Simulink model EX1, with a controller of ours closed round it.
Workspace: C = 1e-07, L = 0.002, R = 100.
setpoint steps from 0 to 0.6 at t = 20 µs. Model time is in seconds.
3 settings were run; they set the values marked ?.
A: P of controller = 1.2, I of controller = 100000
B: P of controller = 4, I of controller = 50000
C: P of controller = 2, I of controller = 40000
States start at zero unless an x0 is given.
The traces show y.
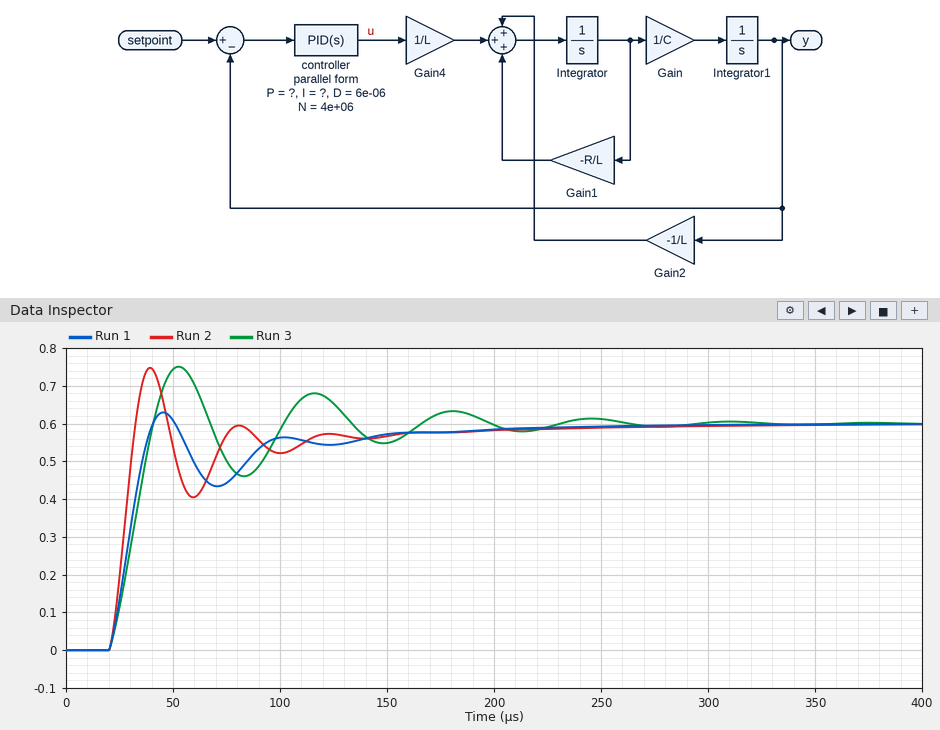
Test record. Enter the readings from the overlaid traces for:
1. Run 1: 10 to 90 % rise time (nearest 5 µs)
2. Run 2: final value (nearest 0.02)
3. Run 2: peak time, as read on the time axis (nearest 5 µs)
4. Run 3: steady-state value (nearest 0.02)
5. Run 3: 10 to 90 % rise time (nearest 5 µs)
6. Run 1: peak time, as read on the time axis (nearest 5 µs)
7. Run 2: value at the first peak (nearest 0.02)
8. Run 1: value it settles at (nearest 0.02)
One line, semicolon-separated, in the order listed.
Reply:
15 µs; 0.60; 40 µs; 0.60; 15 µs; 45 µs; 0.74; 0.60
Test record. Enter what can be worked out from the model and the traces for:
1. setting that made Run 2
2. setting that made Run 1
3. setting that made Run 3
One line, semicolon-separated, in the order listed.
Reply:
B; C; A
